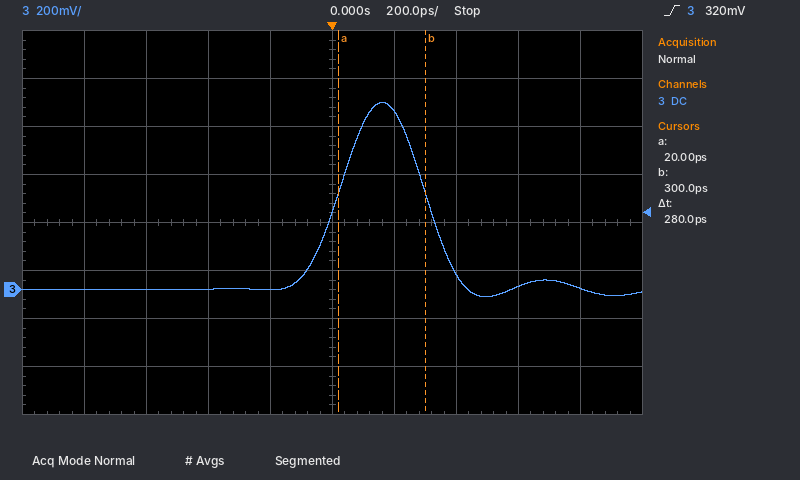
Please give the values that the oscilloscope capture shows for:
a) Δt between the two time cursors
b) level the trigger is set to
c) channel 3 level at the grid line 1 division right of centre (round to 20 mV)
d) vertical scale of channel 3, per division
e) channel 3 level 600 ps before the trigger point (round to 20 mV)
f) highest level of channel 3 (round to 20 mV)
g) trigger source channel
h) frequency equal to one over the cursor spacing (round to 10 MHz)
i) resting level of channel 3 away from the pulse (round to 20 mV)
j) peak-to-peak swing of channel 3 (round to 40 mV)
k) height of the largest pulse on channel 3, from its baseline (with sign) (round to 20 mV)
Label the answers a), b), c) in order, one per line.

a) 280 ps
b) 320 mV
c) 740 mV
d) 200 mV
e) 0 mV
f) 780 mV
g) channel 3
h) 3.57 GHz
i) 0 mV
j) 800 mV
k) +780 mV
